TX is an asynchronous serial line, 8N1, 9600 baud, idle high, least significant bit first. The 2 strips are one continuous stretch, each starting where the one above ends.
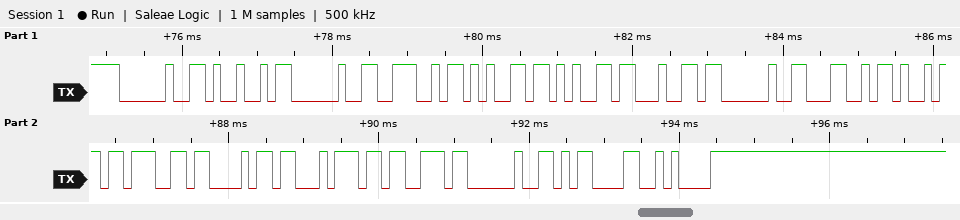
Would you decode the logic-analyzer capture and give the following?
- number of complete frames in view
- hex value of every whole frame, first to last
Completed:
17
20 49 20 4E 65 65 64 20 4C 69 67 68 74 73 20 0D 0A
